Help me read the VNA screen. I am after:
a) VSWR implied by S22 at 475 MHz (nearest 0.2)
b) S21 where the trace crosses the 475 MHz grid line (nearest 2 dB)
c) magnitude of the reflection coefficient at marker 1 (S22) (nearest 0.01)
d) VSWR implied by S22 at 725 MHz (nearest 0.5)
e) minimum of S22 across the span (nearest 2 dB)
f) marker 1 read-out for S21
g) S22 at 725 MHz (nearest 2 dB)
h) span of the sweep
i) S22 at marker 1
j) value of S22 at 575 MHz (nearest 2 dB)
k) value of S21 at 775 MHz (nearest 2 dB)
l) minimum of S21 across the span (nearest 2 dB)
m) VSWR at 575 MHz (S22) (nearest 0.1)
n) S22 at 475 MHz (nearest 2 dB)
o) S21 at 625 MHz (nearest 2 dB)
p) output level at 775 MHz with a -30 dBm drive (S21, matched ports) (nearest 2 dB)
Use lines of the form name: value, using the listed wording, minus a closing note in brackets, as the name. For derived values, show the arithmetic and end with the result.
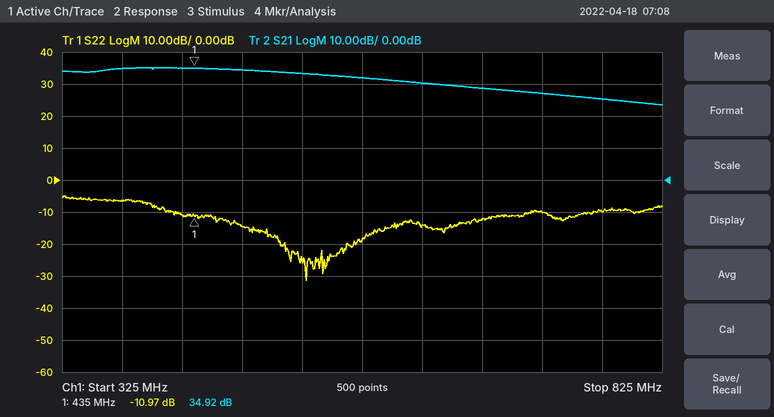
VSWR implied by S22 at 475 MHz: |Γ| = 10^(-14/20) = 0.1995; VSWR = (1 + 0.1995)/(1 − 0.1995) ≈ 1.50, so 1.4 to the nearest 0.2
S21 where the trace crosses the 475 MHz grid line: 34 dB
magnitude of the reflection coefficient at marker 1 (S22): 10^(-10.97/20) ≈ 0.28
VSWR implied by S22 at 725 MHz: |Γ| = 10^(-10/20) = 0.3162; VSWR = (1 + 0.3162)/(1 − 0.3162) ≈ 1.92, so 2.0 to the nearest 0.5
minimum of S22 across the span: -32 dB
marker 1 read-out for S21: 34.92 dB
S22 at 725 MHz: -10 dB
span of the sweep: 500 MHz
S22 at marker 1: -10.97 dB
value of S22 at 575 MHz: -18 dB
value of S21 at 775 MHz: 26 dB
minimum of S21 across the span: 24 dB
VSWR at 575 MHz (S22): |Γ| = 10^(-18/20) = 0.1259; VSWR = (1 + 0.1259)/(1 − 0.1259) ≈ 1.3
S22 at 475 MHz: -14 dB
S21 at 625 MHz: 30 dB
output level at 775 MHz with a -30 dBm drive (S21, matched ports): -30 dBm + (26 dB) = -4 dBm
